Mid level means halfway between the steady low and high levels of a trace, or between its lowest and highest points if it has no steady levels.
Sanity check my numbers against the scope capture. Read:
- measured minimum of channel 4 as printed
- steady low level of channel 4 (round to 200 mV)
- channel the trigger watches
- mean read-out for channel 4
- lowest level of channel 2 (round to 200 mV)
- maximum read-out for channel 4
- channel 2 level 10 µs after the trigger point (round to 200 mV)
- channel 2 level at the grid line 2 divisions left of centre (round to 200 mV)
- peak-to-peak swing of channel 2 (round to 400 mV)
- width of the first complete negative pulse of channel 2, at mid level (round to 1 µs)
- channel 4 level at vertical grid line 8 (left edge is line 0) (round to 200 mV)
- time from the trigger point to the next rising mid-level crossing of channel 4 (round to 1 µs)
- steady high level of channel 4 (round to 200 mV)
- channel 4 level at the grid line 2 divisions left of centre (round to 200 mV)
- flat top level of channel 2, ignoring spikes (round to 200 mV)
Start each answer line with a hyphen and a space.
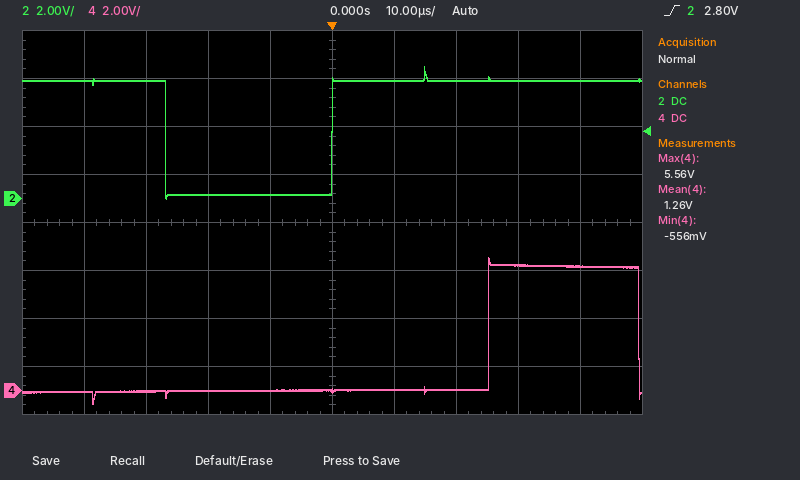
- -556 mV
- 0.0 V
- channel 2
- 1.26 V
- 0.0 V
- 5.56 V
- 5.0 V
- 200 mV
- 5.6 V
- 27 µs
- 5.2 V
- 25 µs
- 5.2 V
- 0.0 V
- 5.0 V
